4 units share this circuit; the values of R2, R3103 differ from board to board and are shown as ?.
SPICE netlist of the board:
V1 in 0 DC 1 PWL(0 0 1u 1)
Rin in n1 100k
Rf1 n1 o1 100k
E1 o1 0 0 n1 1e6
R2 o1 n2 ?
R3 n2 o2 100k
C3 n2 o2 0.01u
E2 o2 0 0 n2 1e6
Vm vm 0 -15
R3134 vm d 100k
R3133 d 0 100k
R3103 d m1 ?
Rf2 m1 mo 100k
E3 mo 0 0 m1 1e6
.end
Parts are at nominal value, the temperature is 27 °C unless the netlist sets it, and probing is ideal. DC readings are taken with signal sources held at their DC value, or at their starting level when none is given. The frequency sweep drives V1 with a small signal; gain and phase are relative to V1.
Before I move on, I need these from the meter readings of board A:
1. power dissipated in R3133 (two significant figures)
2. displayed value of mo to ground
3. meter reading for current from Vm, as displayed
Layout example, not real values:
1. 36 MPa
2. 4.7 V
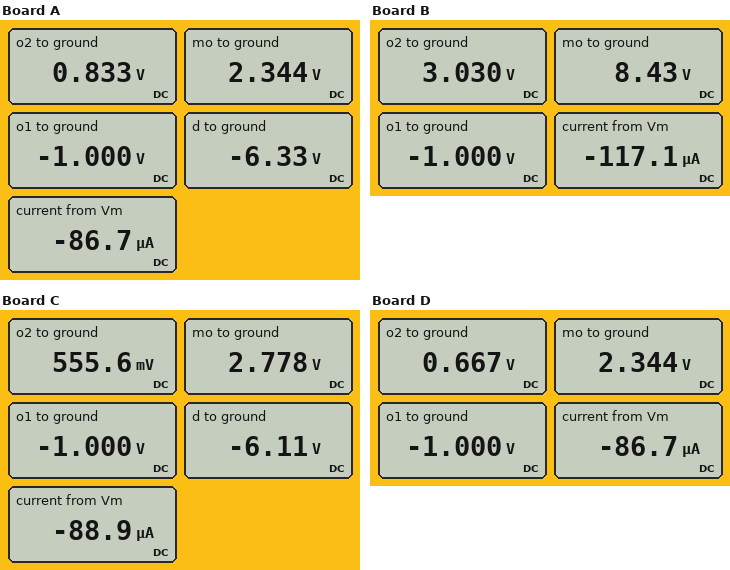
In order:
1. 400 µW
2. 2.344 V
3. -86.7 µA
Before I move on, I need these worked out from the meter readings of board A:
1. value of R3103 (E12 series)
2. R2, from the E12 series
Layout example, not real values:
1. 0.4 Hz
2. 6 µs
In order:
1. 270 kΩ
2. 120 kΩ
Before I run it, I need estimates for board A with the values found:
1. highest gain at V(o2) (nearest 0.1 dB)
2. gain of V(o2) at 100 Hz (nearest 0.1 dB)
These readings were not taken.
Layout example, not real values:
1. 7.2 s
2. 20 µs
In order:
1. -1.6 dB
2. -3.0 dB
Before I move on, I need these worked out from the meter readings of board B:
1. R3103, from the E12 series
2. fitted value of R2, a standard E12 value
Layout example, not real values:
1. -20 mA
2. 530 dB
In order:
1. 39 kΩ
2. 33 kΩ
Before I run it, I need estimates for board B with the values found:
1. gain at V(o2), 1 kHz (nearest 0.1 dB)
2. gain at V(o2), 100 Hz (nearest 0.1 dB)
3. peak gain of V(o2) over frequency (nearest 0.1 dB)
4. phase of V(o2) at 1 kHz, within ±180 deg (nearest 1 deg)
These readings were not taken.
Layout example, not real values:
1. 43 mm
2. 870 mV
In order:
1. -6.4 dB
2. 8.2 dB
3. 9.6 dB
4. -81 deg
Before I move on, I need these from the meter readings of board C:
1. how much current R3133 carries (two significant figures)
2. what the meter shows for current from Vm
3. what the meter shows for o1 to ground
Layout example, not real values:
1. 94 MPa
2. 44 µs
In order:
1. 61 µA
2. -88.9 µA
3. -1.000 V
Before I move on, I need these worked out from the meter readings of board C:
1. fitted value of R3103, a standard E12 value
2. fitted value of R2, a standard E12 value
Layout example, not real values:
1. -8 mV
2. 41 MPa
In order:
1. 220 kΩ
2. 180 kΩ
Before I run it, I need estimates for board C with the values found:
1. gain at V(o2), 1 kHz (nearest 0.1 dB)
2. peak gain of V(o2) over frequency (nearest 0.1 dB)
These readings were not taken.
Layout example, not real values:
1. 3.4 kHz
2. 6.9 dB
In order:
1. -21.2 dB
2. -5.1 dB
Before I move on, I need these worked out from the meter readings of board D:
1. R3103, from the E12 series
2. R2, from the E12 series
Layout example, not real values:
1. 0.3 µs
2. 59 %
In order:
1. 270 kΩ
2. 150 kΩ
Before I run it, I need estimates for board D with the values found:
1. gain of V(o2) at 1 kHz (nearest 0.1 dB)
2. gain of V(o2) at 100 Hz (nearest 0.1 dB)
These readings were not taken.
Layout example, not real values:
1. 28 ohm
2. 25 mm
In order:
1. -19.6 dB
2. -5.0 dB
